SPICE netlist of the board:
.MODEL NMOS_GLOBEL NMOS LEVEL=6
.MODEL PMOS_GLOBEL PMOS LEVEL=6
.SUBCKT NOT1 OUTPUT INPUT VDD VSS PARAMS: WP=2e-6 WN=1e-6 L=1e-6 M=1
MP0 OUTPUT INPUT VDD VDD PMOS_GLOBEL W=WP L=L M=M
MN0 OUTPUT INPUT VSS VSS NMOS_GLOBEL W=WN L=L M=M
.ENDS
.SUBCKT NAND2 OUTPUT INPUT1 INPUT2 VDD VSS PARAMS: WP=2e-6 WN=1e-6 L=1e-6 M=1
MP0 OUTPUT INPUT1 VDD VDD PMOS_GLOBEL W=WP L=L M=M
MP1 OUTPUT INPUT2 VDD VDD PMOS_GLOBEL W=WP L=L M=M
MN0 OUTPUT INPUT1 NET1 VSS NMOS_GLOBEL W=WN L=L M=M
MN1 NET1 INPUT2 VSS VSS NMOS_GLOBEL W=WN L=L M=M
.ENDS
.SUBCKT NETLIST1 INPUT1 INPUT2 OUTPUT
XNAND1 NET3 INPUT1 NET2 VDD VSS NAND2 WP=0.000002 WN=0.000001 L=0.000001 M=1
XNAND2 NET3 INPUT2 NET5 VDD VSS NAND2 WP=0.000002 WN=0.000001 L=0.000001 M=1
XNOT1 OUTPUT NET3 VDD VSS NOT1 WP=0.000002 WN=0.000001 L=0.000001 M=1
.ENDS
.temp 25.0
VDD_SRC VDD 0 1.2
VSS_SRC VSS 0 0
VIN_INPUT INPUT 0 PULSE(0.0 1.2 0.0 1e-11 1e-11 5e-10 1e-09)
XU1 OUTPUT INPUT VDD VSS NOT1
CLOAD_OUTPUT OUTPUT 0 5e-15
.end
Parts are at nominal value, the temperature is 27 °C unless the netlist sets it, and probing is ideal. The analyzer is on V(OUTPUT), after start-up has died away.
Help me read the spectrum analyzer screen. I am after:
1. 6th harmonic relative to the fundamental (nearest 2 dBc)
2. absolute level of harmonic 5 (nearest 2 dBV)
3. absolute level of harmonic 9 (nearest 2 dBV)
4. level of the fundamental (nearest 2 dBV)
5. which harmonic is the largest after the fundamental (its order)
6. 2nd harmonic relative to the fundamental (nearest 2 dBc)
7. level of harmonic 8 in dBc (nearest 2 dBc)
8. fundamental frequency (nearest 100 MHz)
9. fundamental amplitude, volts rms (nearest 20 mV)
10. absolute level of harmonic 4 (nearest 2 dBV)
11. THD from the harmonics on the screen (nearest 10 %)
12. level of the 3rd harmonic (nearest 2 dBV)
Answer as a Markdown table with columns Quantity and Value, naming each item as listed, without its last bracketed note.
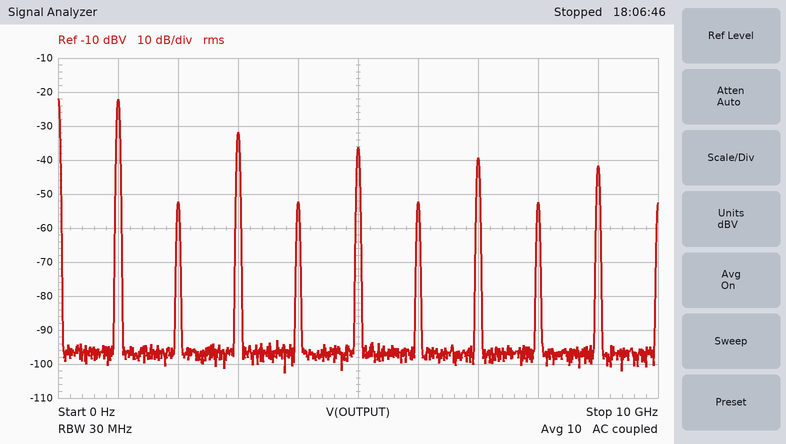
| Quantity | Value |
|---|---|
| 6th harmonic relative to the fundamental | -30 dBc |
| absolute level of harmonic 5 | -36 dBV |
| absolute level of harmonic 9 | -42 dBV |
| level of the fundamental | -22 dBV |
| which harmonic is the largest after the fundamental | 3 |
| 2nd harmonic relative to the fundamental | -30 dBc |
| level of harmonic 8 in dBc | -30 dBc |
| fundamental frequency | 1.0 GHz |
| fundamental amplitude, volts rms | 80 mV |
| absolute level of harmonic 4 | -52 dBV |
| THD from the harmonics on the screen | 40 % |
| level of the 3rd harmonic | -32 dBV |
